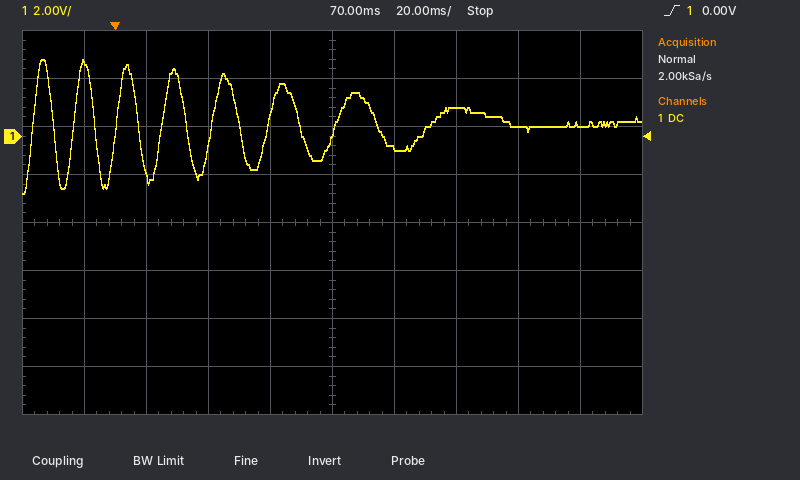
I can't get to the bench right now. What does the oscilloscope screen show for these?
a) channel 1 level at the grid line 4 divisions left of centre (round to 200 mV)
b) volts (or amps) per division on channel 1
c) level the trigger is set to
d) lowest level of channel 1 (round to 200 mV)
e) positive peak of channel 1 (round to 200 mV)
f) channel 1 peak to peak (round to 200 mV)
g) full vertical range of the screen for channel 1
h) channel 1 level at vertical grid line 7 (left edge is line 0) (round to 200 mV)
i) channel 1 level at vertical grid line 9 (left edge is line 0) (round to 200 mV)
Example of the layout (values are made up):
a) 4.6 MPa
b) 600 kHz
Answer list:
a) 3.0 V
b) 2 V
c) 0.00 V
d) -2.4 V
e) 3.2 V
f) 5.6 V
g) 16 V
h) 1.2 V
i) 400 mV
